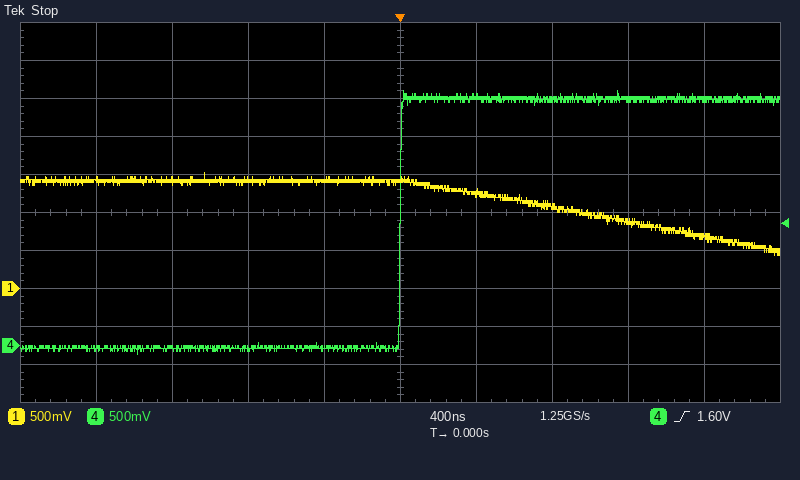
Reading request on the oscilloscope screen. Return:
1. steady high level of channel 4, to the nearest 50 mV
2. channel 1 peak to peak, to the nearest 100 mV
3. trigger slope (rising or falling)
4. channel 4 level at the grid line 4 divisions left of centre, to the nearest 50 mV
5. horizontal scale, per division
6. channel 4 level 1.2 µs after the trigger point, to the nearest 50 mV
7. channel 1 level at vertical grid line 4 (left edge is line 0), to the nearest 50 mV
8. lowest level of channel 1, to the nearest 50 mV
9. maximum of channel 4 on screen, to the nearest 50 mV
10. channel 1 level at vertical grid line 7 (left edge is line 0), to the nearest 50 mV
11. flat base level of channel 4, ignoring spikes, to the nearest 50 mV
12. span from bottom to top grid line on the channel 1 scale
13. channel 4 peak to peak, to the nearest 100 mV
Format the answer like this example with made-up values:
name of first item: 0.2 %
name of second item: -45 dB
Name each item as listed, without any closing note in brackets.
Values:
steady high level of channel 4, to the nearest 50 mV: 3.25 V
channel 1 peak to peak, to the nearest 100 mV: 1.10 V
trigger slope: rising
channel 4 level at the grid line 4 divisions left of centre, to the nearest 50 mV: -50 mV
horizontal scale, per division: 400 ns
channel 4 level 1.2 µs after the trigger point, to the nearest 50 mV: 3.25 V
channel 1 level at vertical grid line 4 (left edge is line 0), to the nearest 50 mV: 1.45 V
lowest level of channel 1, to the nearest 50 mV: 450 mV
maximum of channel 4 on screen, to the nearest 50 mV: 3.35 V
channel 1 level at vertical grid line 7 (left edge is line 0), to the nearest 50 mV: 1.10 V
flat base level of channel 4, ignoring spikes, to the nearest 50 mV: -50 mV
span from bottom to top grid line on the channel 1 scale: 5 V
channel 4 peak to peak, to the nearest 100 mV: 3.50 V
